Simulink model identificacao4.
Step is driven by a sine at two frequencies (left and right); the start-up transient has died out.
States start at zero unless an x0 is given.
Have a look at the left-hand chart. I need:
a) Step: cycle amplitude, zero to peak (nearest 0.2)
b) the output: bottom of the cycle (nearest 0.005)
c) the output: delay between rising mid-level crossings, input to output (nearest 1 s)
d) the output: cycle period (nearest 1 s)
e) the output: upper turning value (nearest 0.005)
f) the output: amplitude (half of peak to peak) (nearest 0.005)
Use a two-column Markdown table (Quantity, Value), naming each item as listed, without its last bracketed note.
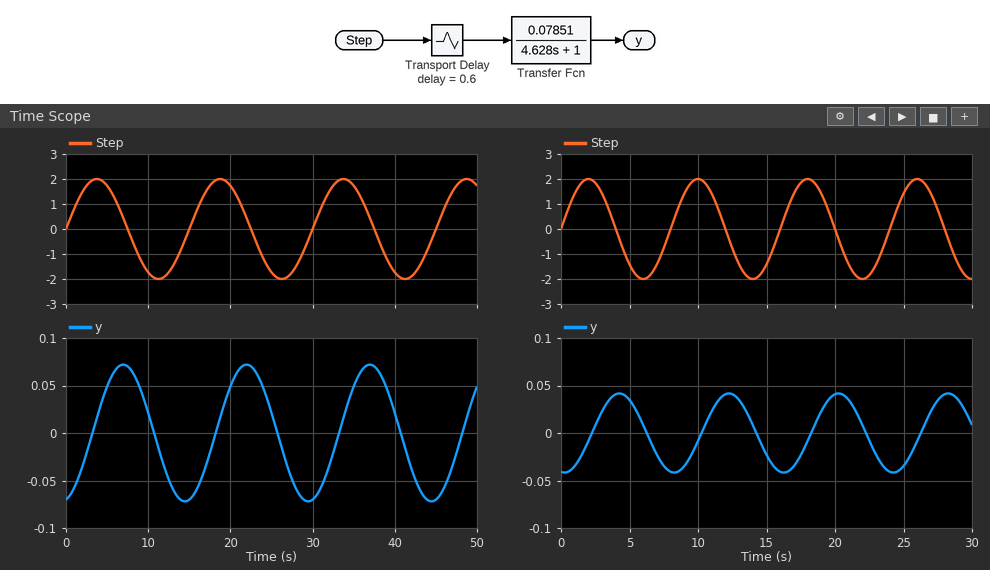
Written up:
| Quantity | Value |
|---|---|
| Step: cycle amplitude, zero to peak | 2.0 |
| the output: bottom of the cycle | -0.070 |
| the output: delay between rising mid-level crossings, input to output | 3 s |
| the output: cycle period | 15 s |
| the output: upper turning value | 0.070 |
| the output: amplitude (half of peak to peak) | 0.070 |
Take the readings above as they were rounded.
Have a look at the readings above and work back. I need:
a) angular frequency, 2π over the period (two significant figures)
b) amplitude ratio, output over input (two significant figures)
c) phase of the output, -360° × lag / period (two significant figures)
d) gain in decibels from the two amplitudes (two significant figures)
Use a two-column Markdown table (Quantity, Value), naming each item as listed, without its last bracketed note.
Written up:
| Quantity | Value |
|---|---|
| angular frequency, 2π over the period | 0.42 rad/s |
| amplitude ratio, output over input | 0.035 |
| phase of the output, -360° × lag / period | -72° |
| gain in decibels from the two amplitudes | -29 dB |
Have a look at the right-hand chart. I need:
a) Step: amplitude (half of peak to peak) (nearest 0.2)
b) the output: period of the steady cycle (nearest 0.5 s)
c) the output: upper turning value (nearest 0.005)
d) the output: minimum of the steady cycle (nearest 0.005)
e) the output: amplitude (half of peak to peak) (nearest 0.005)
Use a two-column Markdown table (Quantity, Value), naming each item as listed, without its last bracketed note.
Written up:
| Quantity | Value |
|---|---|
| Step: amplitude (half of peak to peak) | 2.0 |
| the output: period of the steady cycle | 8.0 s |
| the output: upper turning value | 0.040 |
| the output: minimum of the steady cycle | -0.040 |
| the output: amplitude (half of peak to peak) | 0.040 |
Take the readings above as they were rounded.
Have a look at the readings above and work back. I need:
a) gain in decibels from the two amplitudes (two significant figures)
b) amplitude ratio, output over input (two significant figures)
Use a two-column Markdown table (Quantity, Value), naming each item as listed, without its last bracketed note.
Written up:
| Quantity | Value |
|---|---|
| gain in decibels from the two amplitudes | -34 dB |
| amplitude ratio, output over input | 0.020 |
